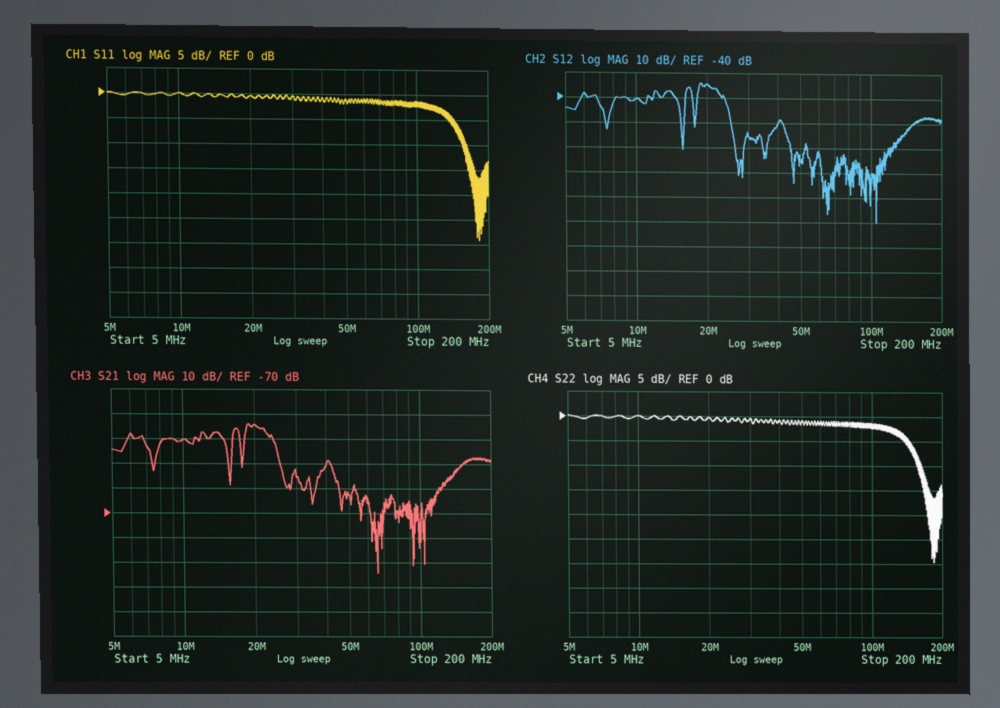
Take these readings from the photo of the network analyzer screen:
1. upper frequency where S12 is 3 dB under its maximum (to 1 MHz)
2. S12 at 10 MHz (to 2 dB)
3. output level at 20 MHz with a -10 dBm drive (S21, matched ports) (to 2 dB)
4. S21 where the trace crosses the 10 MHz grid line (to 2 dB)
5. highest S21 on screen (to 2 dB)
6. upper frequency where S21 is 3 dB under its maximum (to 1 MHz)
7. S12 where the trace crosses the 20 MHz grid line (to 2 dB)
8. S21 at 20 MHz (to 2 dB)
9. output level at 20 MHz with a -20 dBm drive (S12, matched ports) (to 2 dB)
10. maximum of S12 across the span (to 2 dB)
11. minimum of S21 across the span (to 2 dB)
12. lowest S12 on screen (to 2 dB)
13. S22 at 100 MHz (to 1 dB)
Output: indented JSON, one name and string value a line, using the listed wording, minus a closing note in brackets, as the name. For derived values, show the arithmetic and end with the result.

{
  "upper frequency where S12 is 3 dB under its maximum": "22 MHz",
  "S12 at 10 MHz": "-40 dB",
  "output level at 20 MHz with a -10 dBm drive (S21, matched ports)": "-10 dBm + (-34 dB) = -44 dBm",
  "S21 where the trace crosses the 10 MHz grid line": "-40 dB",
  "highest S21 on screen": "-34 dB",
  "upper frequency where S21 is 3 dB under its maximum": "22 MHz",
  "S12 where the trace crosses the 20 MHz grid line": "-34 dB",
  "S21 at 20 MHz": "-34 dB",
  "output level at 20 MHz with a -20 dBm drive (S12, matched ports)": "-20 dBm + (-34 dB) = -54 dBm",
  "maximum of S12 across the span": "-34 dB",
  "minimum of S21 across the span": "-94 dB",
  "lowest S12 on screen": "-90 dB",
  "S22 at 100 MHz": "-2 dB"
}
